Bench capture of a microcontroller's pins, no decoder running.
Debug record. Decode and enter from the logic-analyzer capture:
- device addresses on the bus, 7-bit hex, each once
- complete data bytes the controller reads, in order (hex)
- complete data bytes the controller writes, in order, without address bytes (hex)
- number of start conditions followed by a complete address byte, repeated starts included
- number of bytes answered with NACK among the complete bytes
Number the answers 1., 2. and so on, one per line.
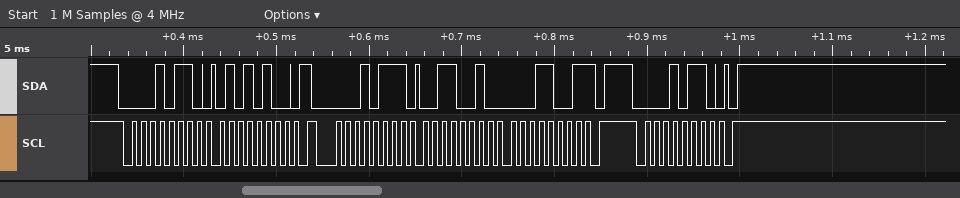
1. 0x0B
2. 32 19
3. 54
4. 3
5. 1
